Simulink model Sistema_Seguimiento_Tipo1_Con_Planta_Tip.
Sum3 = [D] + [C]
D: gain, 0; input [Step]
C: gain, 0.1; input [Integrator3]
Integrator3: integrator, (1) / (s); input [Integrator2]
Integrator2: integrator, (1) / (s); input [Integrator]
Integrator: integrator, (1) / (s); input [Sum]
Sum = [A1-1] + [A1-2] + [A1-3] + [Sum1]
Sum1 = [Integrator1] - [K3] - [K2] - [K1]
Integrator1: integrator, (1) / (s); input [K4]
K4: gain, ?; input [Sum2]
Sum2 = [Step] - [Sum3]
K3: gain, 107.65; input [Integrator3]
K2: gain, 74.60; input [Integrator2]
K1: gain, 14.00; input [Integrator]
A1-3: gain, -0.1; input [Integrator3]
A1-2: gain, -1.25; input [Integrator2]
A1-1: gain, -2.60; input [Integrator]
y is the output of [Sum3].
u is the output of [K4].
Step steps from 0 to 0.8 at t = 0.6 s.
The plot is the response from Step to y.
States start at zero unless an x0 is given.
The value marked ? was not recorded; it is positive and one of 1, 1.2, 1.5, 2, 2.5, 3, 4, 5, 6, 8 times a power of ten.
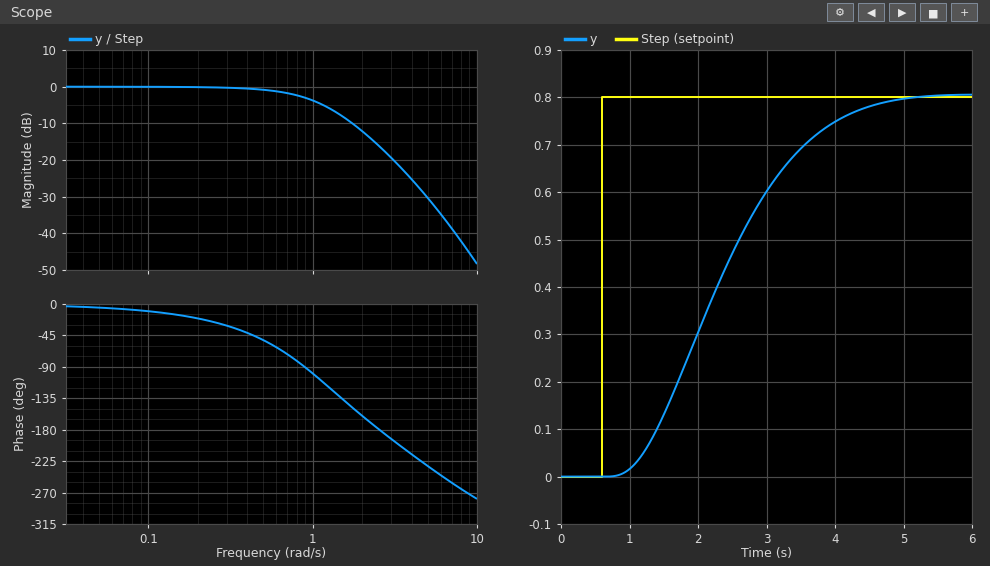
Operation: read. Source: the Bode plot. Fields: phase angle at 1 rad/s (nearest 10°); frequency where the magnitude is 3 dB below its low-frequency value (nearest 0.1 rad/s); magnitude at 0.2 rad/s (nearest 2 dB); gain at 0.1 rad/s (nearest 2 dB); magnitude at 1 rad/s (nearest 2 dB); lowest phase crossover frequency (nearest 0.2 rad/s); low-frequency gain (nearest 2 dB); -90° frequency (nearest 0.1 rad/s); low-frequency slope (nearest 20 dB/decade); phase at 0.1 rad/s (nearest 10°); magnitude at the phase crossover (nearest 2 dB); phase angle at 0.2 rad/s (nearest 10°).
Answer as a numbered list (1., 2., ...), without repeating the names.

1. -100°
2. 0.9 rad/s
3. 0 dB
4. 0 dB
5. -4 dB
6. 2.6 rad/s
7. 0 dB
8. 0.9 rad/s
9. 0 dB/decade
10. -10°
11. -16 dB
12. -20°
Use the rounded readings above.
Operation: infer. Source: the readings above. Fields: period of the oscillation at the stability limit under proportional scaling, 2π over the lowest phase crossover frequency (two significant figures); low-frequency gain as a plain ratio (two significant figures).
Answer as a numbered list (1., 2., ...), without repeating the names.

1. 2.4 s
2. 1.0
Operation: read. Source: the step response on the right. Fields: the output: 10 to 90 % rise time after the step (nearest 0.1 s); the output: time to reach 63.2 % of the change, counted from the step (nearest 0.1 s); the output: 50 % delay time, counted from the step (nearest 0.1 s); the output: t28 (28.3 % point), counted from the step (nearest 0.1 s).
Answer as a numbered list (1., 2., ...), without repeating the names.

1. 2.4 s
2. 2.0 s
3. 1.7 s
4. 1.2 s
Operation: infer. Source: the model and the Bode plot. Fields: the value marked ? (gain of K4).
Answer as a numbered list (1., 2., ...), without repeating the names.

1. 600
